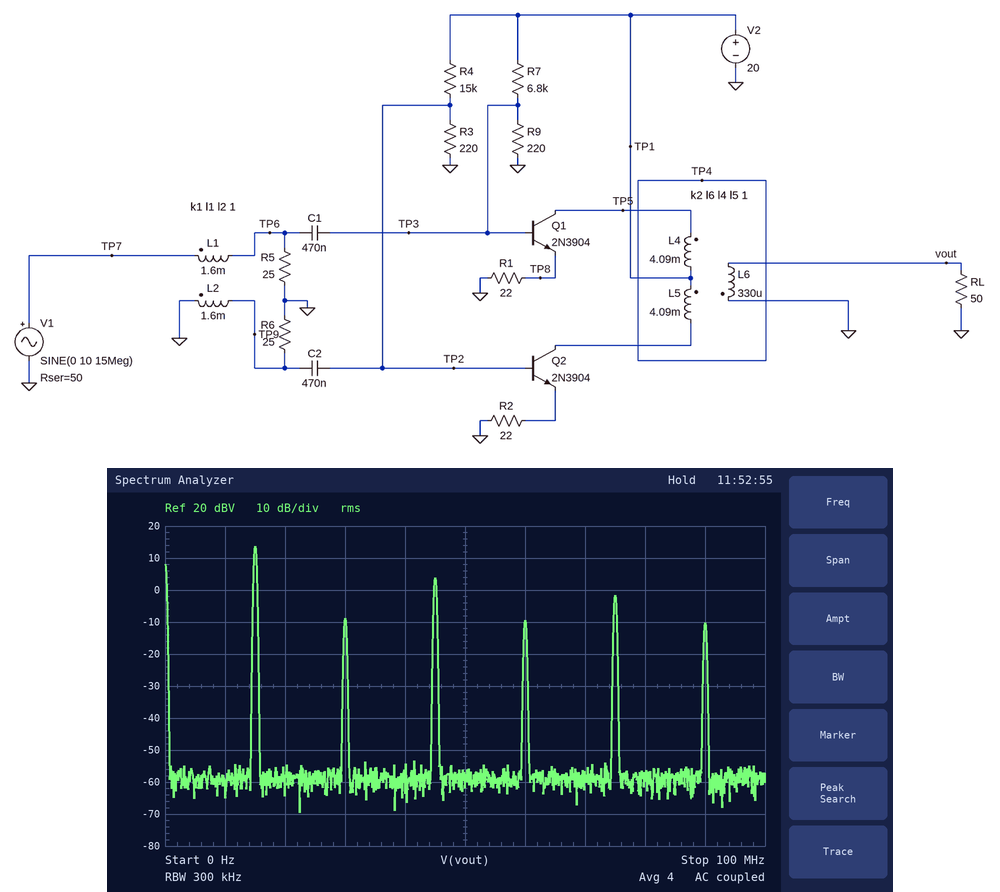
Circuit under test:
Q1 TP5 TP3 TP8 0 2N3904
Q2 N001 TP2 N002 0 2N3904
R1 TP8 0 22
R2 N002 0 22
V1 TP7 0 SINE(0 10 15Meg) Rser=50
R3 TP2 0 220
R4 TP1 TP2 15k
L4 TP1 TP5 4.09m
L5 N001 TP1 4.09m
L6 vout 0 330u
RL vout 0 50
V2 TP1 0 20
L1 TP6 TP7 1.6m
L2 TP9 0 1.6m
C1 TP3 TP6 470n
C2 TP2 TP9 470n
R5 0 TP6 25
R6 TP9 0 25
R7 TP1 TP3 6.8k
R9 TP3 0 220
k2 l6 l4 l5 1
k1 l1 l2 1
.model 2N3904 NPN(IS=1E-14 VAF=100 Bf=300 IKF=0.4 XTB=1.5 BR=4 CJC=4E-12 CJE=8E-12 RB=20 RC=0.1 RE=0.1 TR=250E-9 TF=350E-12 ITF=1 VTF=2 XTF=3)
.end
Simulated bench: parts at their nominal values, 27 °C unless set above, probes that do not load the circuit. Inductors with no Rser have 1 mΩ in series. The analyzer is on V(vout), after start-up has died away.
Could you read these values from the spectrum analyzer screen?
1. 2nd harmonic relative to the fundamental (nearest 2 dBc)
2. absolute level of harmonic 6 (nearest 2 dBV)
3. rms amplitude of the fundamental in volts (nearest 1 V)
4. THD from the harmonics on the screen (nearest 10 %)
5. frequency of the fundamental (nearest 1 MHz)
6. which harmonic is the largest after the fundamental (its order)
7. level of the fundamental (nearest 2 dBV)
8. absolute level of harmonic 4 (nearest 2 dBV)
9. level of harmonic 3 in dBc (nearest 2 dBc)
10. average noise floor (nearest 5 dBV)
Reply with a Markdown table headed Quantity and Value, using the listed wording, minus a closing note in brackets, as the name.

| Quantity | Value |
|---|---|
| 2nd harmonic relative to the fundamental | -22 dBc |
| absolute level of harmonic 6 | -10 dBV |
| rms amplitude of the fundamental in volts | 5 V |
| THD from the harmonics on the screen | 40 % |
| frequency of the fundamental | 15 MHz |
| which harmonic is the largest after the fundamental | 3 |
| level of the fundamental | 14 dBV |
| absolute level of harmonic 4 | -10 dBV |
| level of harmonic 3 in dBc | -10 dBc |
| average noise floor | -60 dBV |
